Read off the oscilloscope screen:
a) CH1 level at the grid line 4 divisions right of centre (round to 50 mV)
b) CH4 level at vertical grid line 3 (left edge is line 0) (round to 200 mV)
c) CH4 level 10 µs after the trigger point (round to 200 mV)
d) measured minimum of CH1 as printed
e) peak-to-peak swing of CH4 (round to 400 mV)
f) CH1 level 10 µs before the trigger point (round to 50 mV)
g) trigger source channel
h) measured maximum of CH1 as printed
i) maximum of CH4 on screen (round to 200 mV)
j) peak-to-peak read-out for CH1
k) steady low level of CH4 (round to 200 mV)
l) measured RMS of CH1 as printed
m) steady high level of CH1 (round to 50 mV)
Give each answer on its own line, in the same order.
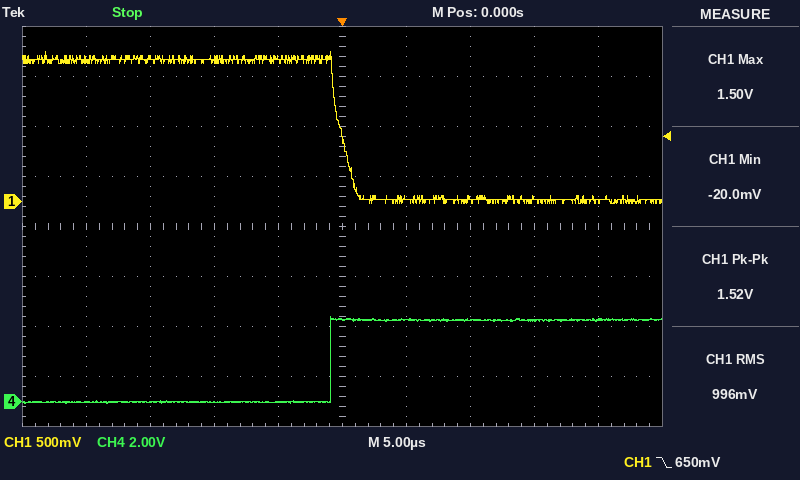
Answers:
0 mV
0.0 V
3.2 V
-20.0 mV
3.6 V
1.40 V
CH1
1.50 V
3.4 V
1.52 V
0.0 V
996 mV
1.40 V
